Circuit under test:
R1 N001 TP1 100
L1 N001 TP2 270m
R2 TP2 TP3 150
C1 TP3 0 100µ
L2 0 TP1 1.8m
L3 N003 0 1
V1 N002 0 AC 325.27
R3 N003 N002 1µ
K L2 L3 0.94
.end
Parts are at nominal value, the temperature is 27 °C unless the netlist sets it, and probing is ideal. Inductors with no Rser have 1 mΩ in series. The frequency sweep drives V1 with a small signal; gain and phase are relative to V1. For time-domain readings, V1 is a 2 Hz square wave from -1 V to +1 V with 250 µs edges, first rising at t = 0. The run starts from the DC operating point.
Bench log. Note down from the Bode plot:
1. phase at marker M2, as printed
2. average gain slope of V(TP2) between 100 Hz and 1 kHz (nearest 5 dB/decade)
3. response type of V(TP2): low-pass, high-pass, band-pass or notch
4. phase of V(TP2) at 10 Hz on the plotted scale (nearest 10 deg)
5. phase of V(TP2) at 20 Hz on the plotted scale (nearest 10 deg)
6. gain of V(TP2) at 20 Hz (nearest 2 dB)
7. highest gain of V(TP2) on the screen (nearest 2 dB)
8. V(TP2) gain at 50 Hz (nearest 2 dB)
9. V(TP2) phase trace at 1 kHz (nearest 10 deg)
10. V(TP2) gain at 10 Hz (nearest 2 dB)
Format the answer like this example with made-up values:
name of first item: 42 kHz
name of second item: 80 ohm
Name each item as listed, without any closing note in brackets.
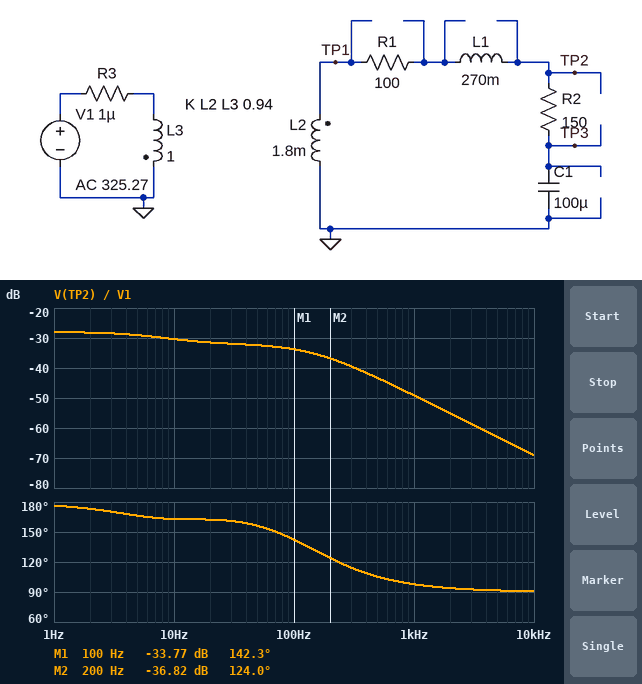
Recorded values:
phase at marker M2, as printed: 124.0 deg
average gain slope of V(TP2) between 100 Hz and 1 kHz: -15 dB/decade
response type of V(TP2): low-pass, high-pass, band-pass or notch: low-pass
phase of V(TP2) at 10 Hz on the plotted scale: 160 deg
phase of V(TP2) at 20 Hz on the plotted scale: 160 deg
gain of V(TP2) at 20 Hz: -32 dB
highest gain of V(TP2) on the screen: -28 dB
V(TP2) gain at 50 Hz: -32 dB
V(TP2) phase trace at 1 kHz: 100 deg
V(TP2) gain at 10 Hz: -30 dB
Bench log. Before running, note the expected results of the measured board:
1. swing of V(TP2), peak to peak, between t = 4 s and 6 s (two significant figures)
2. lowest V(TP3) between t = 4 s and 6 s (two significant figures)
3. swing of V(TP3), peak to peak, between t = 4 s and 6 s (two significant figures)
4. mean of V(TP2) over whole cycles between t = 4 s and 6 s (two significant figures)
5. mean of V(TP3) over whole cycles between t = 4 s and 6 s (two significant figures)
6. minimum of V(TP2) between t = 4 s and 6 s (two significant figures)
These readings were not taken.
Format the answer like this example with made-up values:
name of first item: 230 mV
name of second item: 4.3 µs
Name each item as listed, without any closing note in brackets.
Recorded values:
swing of V(TP2), peak to peak, between t = 4 s and 6 s: 80 mV
lowest V(TP3) between t = 4 s and 6 s: -80 mV
swing of V(TP3), peak to peak, between t = 4 s and 6 s: 80 mV
mean of V(TP2) over whole cycles between t = 4 s and 6 s: -40 mV
mean of V(TP3) over whole cycles between t = 4 s and 6 s: -40 mV
minimum of V(TP2) between t = 4 s and 6 s: -80 mV
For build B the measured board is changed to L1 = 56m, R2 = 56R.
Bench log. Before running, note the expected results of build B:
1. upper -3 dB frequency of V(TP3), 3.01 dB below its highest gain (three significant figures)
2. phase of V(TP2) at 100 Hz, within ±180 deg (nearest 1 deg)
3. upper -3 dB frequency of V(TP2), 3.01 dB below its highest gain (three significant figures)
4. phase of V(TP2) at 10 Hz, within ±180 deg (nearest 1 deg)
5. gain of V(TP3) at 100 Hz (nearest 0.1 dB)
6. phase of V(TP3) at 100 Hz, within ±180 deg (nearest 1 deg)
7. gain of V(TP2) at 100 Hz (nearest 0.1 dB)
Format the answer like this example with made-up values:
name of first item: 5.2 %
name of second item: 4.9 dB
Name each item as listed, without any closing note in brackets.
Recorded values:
upper -3 dB frequency of V(TP3), 3.01 dB below its highest gain: 10.4 Hz
phase of V(TP2) at 100 Hz, within ±180 deg: 157 deg
upper -3 dB frequency of V(TP2), 3.01 dB below its highest gain: 12.2 Hz
phase of V(TP2) at 10 Hz, within ±180 deg: 154 deg
gain of V(TP3) at 100 Hz: -47.9 dB
phase of V(TP3) at 100 Hz, within ±180 deg: 83 deg
gain of V(TP2) at 100 Hz: -36.6 dB
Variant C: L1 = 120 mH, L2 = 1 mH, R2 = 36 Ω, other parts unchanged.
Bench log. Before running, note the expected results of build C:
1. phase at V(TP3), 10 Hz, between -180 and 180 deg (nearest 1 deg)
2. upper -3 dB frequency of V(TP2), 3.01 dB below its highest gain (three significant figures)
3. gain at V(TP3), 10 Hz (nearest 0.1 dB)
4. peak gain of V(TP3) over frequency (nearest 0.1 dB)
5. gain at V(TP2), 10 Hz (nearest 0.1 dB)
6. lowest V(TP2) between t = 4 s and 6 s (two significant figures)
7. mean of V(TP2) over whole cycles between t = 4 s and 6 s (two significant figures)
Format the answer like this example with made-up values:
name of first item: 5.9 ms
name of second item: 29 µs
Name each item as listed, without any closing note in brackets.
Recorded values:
phase at V(TP3), 10 Hz, between -180 and 180 deg: 138 deg
upper -3 dB frequency of V(TP2), 3.01 dB below its highest gain: 13.6 Hz
gain at V(TP3), 10 Hz: -32.7 dB
peak gain of V(TP3) over frequency: -30.5 dB
gain at V(TP2), 10 Hz: -32.5 dB
lowest V(TP2) between t = 4 s and 6 s: -59 mV
mean of V(TP2) over whole cycles between t = 4 s and 6 s: -30 mV
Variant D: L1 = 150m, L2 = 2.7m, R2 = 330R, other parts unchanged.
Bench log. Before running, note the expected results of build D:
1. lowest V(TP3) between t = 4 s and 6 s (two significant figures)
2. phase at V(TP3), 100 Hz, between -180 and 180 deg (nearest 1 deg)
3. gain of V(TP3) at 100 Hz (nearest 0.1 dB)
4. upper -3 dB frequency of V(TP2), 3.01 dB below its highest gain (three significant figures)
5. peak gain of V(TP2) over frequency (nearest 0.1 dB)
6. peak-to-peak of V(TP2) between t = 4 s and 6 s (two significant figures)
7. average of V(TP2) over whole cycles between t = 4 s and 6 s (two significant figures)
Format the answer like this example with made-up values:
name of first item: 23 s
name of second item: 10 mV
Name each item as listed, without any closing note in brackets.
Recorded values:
lowest V(TP3) between t = 4 s and 6 s: -97 mV
phase at V(TP3), 100 Hz, between -180 and 180 deg: 80 deg
gain of V(TP3) at 100 Hz: -55.0 dB
upper -3 dB frequency of V(TP2), 3.01 dB below its highest gain: 201 Hz
peak gain of V(TP2) over frequency: -26.2 dB
peak-to-peak of V(TP2) between t = 4 s and 6 s: 98 mV
average of V(TP2) over whole cycles between t = 4 s and 6 s: -49 mV
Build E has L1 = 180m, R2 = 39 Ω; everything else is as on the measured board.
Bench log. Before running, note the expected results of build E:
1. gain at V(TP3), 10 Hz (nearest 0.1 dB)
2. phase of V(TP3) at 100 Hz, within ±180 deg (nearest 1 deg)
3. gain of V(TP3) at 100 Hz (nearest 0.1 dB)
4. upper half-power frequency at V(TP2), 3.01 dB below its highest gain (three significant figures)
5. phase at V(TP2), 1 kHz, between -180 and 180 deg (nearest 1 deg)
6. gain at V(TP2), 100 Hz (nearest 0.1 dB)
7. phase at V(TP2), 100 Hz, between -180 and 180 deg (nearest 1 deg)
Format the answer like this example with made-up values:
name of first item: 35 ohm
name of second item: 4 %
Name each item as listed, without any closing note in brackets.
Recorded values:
gain at V(TP3), 10 Hz: -30.1 dB
phase of V(TP3) at 100 Hz, within ±180 deg: 55 deg
gain of V(TP3) at 100 Hz: -48.5 dB
upper half-power frequency at V(TP2), 3.01 dB below its highest gain: 14.0 Hz
phase at V(TP2), 1 kHz, between -180 and 180 deg: 95 deg
gain at V(TP2), 100 Hz: -40.1 dB
phase at V(TP2), 100 Hz, between -180 and 180 deg: 123 deg
